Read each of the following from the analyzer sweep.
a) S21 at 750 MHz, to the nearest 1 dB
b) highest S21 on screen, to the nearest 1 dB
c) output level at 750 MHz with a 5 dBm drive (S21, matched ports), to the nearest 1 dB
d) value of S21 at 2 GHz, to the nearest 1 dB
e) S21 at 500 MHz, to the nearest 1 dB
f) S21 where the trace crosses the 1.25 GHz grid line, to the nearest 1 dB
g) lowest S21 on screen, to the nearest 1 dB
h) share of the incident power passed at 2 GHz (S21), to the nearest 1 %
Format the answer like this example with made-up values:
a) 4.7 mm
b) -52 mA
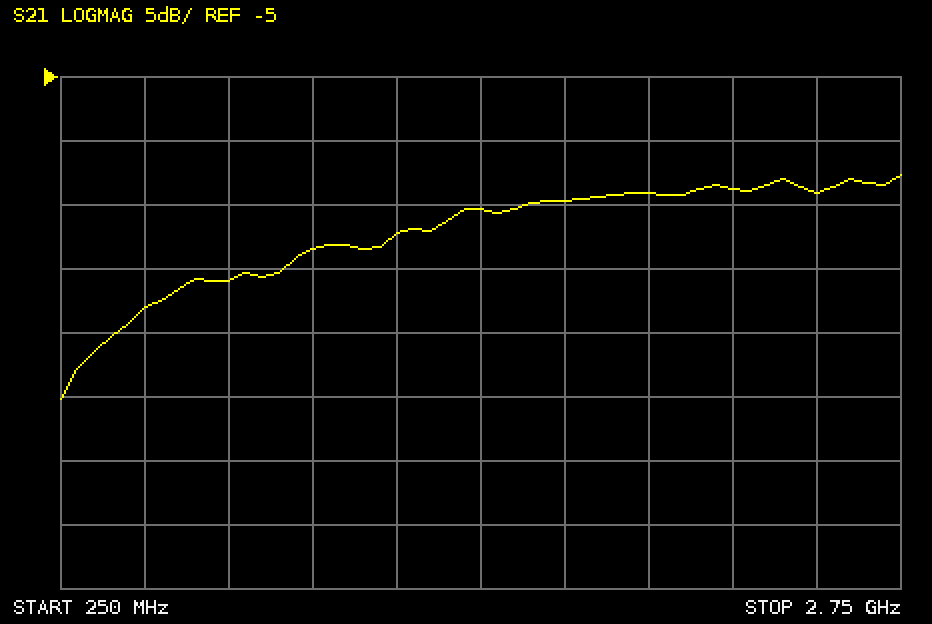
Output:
a) -21 dB
b) -13 dB
c) -16 dBm
d) -14 dB
e) -23 dB
f) -17 dB
g) -30 dB
h) 4 %
